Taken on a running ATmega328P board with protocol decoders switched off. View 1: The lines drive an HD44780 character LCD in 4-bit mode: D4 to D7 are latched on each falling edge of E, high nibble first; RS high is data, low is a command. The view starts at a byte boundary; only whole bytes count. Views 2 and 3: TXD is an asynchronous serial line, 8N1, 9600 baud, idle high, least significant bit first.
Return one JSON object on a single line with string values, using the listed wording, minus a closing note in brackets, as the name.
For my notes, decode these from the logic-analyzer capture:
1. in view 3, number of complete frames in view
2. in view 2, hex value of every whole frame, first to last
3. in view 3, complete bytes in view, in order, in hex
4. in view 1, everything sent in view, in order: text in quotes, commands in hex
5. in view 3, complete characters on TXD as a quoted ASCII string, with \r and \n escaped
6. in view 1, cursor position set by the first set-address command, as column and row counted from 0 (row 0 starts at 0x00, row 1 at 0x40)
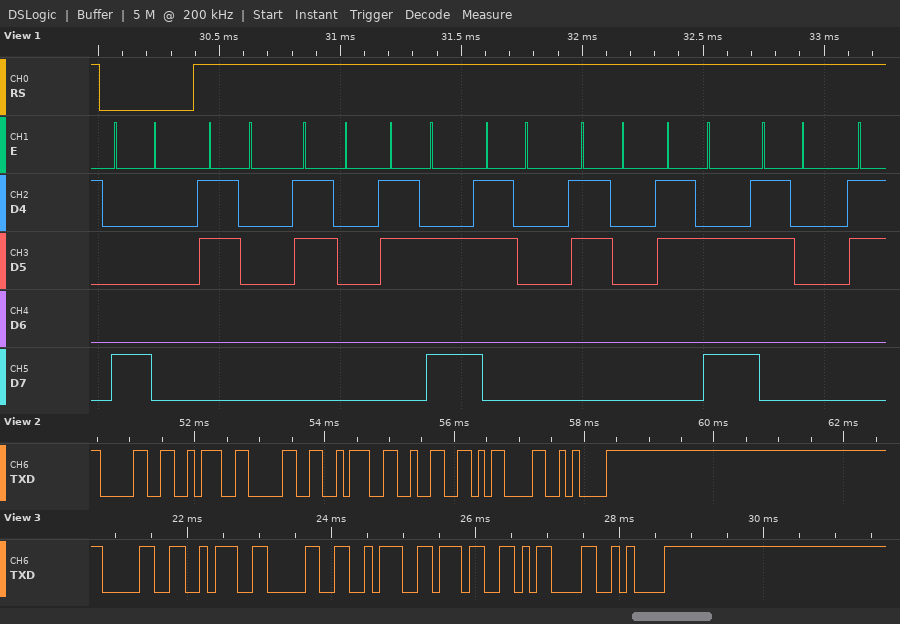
{"in view 3, number of complete frames in view": "7", "in view 2, hex value of every whole frame, first to last": "30 3A 30 3A 32 0D 0A", "in view 3, complete bytes in view, in order, in hex": "0x30 0x3A 0x30 0x3A 0x37 0x0D 0x0A", "in view 1, everything sent in view, in order: text in quotes, commands in hex": "0x80 \"00:00:0\"", "in view 3, complete characters on TXD as a quoted ASCII string, with \\r and \\n escaped": "\"0:0:7\\r\\n\"", "in view 1, cursor position set by the first set-address command, as column and row counted from 0": "column 0, row 0"}
